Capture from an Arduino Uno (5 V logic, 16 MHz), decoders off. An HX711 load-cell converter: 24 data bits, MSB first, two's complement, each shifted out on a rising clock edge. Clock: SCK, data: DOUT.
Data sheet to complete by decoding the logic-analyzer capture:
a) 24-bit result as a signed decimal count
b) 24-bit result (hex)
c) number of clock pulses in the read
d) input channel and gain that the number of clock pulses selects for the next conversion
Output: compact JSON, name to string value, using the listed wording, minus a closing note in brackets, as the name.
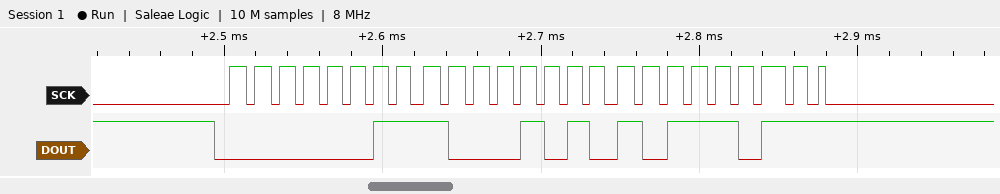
{"24-bit result as a signed decimal count": "232123", "24-bit result": "0x038ABB", "number of clock pulses in the read": "25", "input channel and gain that the number of clock pulses selects for the next conversion": "channel A, gain 128"}
